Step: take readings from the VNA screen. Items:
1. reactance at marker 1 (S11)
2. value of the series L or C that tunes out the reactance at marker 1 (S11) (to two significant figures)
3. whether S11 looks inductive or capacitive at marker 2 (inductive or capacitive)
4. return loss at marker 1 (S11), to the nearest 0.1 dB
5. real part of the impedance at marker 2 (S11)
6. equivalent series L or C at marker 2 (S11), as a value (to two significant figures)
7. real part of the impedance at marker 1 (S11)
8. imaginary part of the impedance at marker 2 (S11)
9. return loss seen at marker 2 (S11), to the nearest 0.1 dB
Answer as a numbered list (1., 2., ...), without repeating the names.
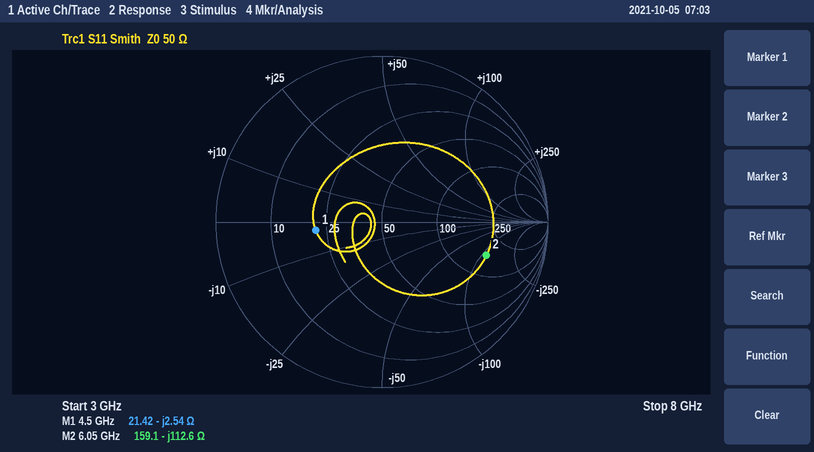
1. -2.54 Ω
2. 90 pH
3. capacitive
4. 7.9 dB
5. 159.1 Ω
6. 230 fF
7. 21.42 Ω
8. -112.6 Ω
9. 3.6 dB
